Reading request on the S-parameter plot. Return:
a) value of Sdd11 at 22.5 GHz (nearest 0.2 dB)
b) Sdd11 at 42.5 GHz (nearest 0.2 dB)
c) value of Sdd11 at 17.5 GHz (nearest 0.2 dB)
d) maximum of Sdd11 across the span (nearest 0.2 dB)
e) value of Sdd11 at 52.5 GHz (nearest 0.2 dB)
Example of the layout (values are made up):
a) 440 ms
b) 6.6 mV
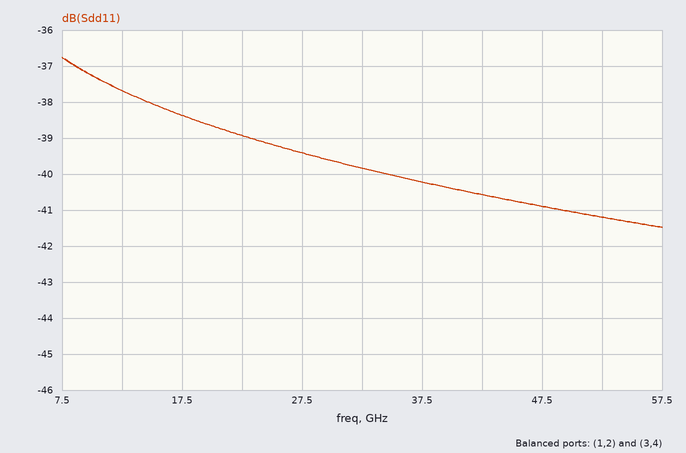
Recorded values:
a) -39.0 dB
b) -40.6 dB
c) -38.4 dB
d) -36.8 dB
e) -41.2 dB
